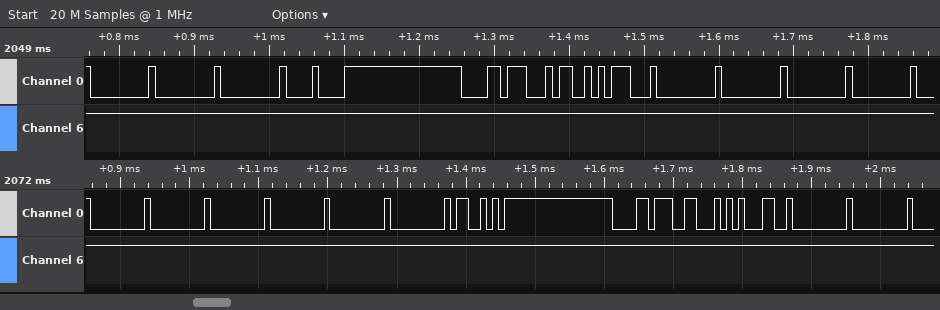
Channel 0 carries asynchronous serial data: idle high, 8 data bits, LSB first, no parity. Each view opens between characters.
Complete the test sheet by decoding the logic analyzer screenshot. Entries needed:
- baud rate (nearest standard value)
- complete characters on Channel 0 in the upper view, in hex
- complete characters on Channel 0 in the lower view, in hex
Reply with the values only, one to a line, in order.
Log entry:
115200 baud
00, 00, 00, 08, D8, 34, 1D, 00, 00, 00, 00
00, 00, 00, 00, 00, 00, 53, D8, 46, 31, 00, 00
